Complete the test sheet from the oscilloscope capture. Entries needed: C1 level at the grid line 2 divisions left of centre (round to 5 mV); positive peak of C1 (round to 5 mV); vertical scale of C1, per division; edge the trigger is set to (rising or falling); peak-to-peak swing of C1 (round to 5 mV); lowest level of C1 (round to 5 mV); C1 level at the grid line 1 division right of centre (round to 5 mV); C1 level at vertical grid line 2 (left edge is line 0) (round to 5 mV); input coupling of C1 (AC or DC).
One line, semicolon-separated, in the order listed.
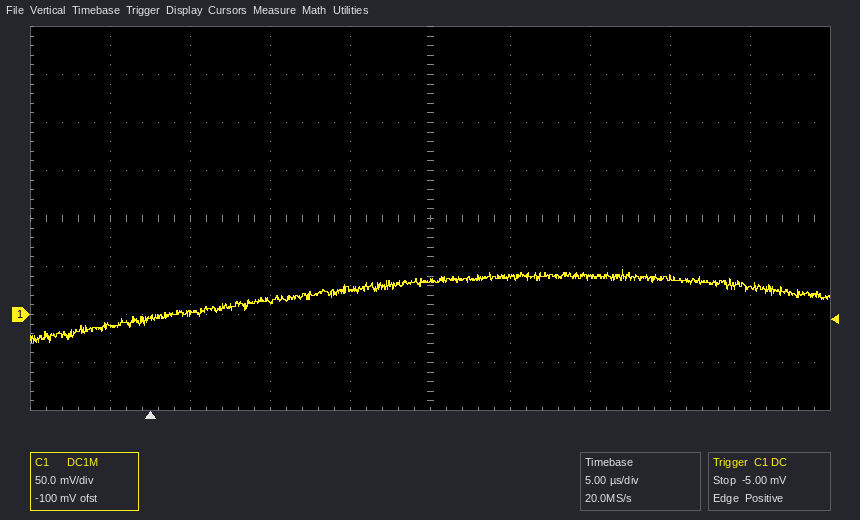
15 mV; 45 mV; 50 mV; rising; 75 mV; -30 mV; 40 mV; 0 mV; DC
